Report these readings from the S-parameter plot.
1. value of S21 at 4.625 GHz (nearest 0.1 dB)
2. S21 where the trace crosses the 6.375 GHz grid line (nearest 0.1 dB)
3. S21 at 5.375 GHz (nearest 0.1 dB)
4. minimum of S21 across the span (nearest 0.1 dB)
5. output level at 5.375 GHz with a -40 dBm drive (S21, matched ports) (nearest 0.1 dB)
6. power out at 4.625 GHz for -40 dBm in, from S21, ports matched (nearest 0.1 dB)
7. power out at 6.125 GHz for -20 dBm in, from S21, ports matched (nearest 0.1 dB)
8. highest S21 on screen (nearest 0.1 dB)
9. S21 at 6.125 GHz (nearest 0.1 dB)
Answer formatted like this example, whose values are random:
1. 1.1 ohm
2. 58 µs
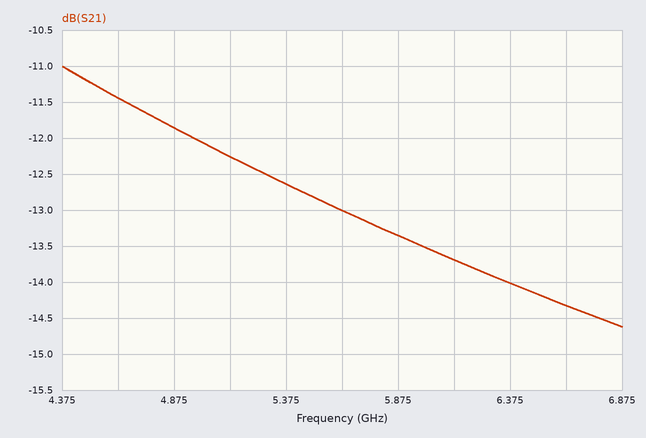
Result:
1. -11.4 dB
2. -14.0 dB
3. -12.6 dB
4. -14.6 dB
5. -52.6 dBm
6. -51.4 dBm
7. -33.7 dBm
8. -11.0 dB
9. -13.7 dB
